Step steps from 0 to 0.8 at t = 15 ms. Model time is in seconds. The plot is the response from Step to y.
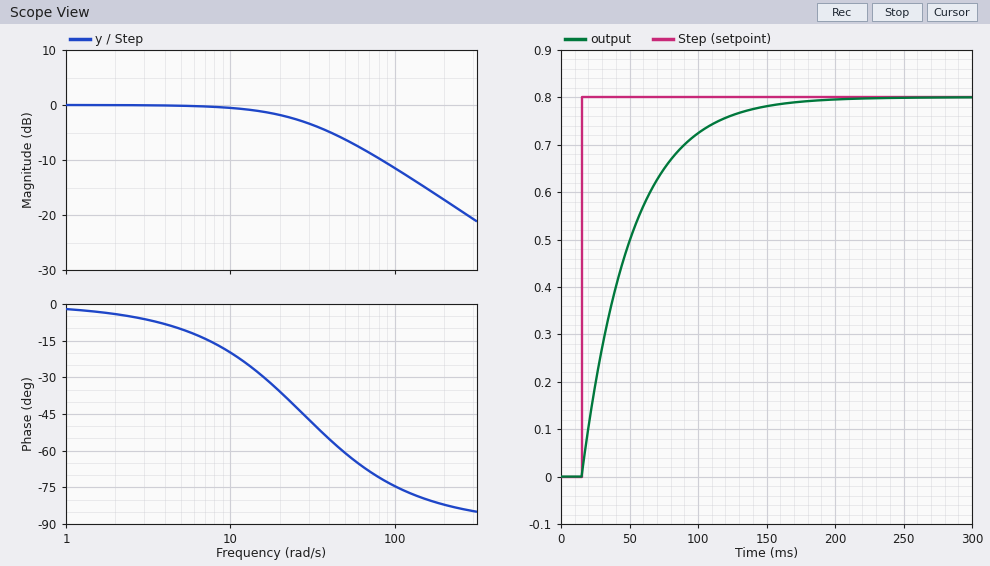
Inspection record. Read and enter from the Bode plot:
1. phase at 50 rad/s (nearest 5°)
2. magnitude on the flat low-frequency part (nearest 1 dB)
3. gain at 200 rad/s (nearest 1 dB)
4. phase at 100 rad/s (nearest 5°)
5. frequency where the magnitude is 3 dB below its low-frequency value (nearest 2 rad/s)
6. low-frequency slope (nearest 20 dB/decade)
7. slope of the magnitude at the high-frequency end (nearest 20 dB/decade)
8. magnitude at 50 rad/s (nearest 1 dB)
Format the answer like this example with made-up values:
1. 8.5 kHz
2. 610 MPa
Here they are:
1. -60°
2. 0 dB
3. -17 dB
4. -75°
5. 28 rad/s
6. 0 dB/decade
7. -20 dB/decade
8. -6 dB
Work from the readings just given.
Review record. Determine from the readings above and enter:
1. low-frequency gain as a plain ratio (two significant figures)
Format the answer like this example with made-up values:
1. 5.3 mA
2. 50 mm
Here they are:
1. 1.0
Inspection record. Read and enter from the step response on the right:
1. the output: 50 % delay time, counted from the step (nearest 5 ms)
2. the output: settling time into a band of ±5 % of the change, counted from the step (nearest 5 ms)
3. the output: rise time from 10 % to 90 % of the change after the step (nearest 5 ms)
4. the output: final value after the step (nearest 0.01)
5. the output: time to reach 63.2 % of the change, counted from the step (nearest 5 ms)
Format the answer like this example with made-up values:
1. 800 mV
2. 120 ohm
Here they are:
1. 25 ms
2. 110 ms
3. 80 ms
4. 0.80
5. 35 ms
